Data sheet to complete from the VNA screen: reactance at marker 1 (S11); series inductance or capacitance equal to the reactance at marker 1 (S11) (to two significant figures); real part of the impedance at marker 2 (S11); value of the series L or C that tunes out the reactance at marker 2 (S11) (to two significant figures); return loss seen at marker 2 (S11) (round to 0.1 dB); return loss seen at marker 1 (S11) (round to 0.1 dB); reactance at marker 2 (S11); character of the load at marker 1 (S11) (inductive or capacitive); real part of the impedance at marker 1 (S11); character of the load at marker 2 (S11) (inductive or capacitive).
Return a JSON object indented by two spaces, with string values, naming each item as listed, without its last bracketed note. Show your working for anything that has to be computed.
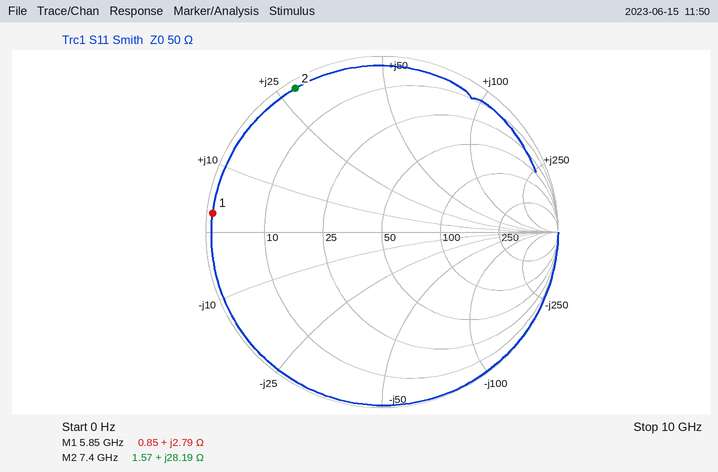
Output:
{
  "reactance at marker 1": "+2.79 Ω",
  "series inductance or capacitance equal to the reactance at marker 1 (S11)": "L = 2.79 Ω/(2π × 5.85 GHz) ≈ 76 pH",
  "real part of the impedance at marker 2": "1.57 Ω",
  "value of the series L or C that tunes out the reactance at marker 2 (S11)": "C = 1/(2π × 7.4 GHz × 28.19 Ω) ≈ 763 fF, so 760 fF to two significant figures",
  "return loss seen at marker 2 (S11)": "0.4 dB",
  "return loss seen at marker 1 (S11)": "0.3 dB",
  "reactance at marker 2": "+28.19 Ω",
  "character of the load at marker 1 (S11)": "inductive",
  "real part of the impedance at marker 1": "0.85 Ω",
  "character of the load at marker 2 (S11)": "inductive"
}
